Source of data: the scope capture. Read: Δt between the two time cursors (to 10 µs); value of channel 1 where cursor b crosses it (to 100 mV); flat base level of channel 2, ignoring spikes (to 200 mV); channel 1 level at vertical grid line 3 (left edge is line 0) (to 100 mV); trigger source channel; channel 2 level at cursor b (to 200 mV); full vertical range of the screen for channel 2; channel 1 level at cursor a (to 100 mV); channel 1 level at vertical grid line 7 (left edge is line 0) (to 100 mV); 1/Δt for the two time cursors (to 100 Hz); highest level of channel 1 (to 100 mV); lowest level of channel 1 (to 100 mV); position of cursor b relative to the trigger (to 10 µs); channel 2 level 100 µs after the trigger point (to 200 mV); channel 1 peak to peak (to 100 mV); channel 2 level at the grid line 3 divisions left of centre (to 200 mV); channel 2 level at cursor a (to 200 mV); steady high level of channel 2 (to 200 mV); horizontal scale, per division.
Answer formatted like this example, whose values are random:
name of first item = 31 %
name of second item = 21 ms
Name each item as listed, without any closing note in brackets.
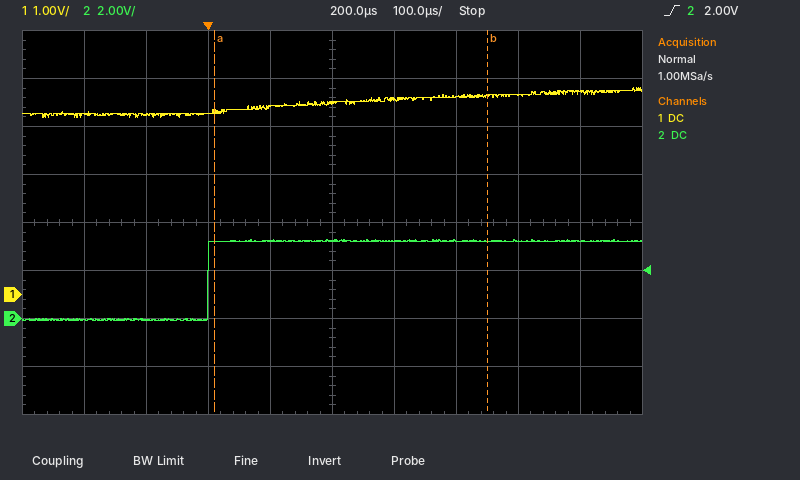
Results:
Δt between the two time cursors = 440 µs
value of channel 1 where cursor b crosses it = 4.1 V
flat base level of channel 2, ignoring spikes = 0.0 V
channel 1 level at vertical grid line 3 (left edge is line 0) = 3.8 V
trigger source channel = channel 2
channel 2 level at cursor b = 3.2 V
full vertical range of the screen for channel 2 = 16 V
channel 1 level at cursor a = 3.8 V
channel 1 level at vertical grid line 7 (left edge is line 0) = 4.1 V
1/Δt for the two time cursors = 2.3 kHz
highest level of channel 1 = 4.3 V
lowest level of channel 1 = 3.7 V
position of cursor b relative to the trigger = +450 µs
channel 2 level 100 µs after the trigger point = 3.2 V
channel 1 peak to peak = 600 mV
channel 2 level at the grid line 3 divisions left of centre = 0.0 V
channel 2 level at cursor a = 3.2 V
steady high level of channel 2 = 3.2 V
horizontal scale, per division = 100 µs
